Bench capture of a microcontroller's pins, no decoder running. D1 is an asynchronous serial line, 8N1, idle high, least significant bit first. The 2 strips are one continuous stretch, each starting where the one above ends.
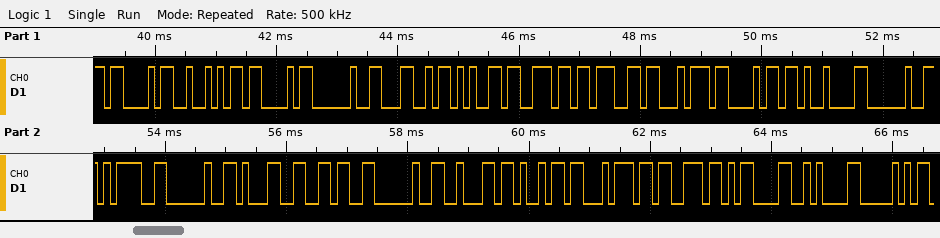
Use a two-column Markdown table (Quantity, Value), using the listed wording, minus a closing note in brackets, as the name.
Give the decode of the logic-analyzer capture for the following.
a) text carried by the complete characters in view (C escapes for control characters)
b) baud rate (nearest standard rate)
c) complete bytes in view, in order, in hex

| Quantity | Value |
|---|---|
| text carried by the complete characters in view | "CRC Length\t = 16 bits\r\nP" |
| baud rate | 9600 baud |
| complete bytes in view, in order, in hex | 43 52 43 20 4C 65 6E 67 74 68 09 20 3D 20 31 36 20 62 69 74 73 0D 0A 50 |
